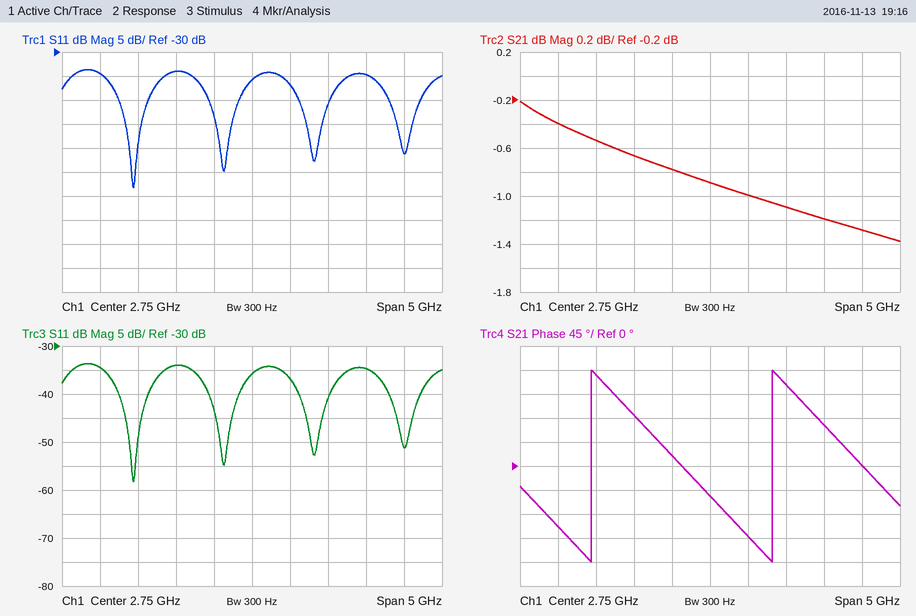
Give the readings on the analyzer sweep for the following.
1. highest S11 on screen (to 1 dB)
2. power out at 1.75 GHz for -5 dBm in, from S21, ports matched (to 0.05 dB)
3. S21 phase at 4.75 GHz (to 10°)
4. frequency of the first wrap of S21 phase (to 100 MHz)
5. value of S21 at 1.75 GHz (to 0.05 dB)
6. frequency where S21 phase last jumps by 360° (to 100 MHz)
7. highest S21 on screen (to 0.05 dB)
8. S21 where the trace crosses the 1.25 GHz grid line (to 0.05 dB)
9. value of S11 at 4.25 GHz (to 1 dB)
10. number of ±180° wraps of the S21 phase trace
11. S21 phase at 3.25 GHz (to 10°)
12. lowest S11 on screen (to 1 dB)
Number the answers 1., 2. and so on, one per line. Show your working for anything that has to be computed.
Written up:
1. -34 dB
2. -5 dBm + (-0.65 dB) = -5.65 dBm
3. 0°
4. 1.2 GHz
5. -0.65 dB
6. 3.6 GHz
7. -0.20 dB
8. -0.55 dB
9. -35 dB
10. 2
11. -130°
12. -58 dB
